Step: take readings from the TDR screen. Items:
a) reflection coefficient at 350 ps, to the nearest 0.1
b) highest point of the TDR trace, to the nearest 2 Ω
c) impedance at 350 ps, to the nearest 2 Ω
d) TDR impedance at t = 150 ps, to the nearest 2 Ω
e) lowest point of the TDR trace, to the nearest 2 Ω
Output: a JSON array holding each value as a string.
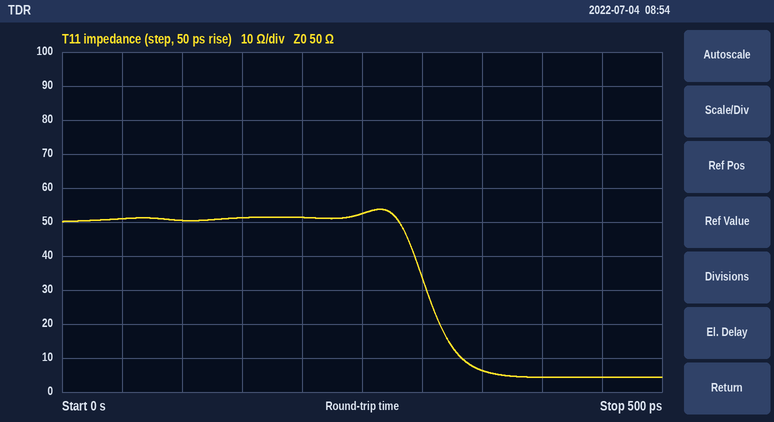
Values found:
["-0.8", "54 Ω", "6 Ω", "52 Ω", "4 Ω"]
